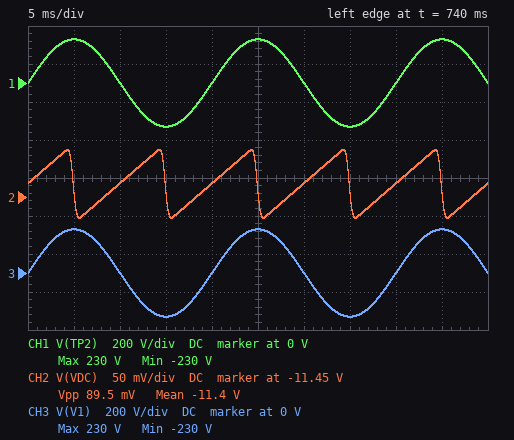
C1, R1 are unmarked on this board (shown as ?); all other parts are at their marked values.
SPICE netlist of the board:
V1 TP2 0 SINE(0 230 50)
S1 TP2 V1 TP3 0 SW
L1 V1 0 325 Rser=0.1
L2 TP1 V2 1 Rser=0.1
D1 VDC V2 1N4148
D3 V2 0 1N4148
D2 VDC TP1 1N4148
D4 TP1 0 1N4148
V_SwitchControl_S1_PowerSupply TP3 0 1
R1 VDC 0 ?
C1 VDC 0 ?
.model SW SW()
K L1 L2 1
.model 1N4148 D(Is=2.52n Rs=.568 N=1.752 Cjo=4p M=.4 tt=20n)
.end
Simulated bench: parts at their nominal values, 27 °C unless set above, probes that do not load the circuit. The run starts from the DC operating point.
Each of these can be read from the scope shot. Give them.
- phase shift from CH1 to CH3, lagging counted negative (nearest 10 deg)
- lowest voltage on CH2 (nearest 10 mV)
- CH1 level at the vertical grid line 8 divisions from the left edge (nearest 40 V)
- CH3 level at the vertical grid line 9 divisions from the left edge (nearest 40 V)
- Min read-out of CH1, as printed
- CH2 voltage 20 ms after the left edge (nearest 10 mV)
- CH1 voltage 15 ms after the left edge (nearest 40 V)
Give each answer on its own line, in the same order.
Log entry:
0 deg
-11.48 V
0 V
240 V
-230 V
-11.43 V
-240 V
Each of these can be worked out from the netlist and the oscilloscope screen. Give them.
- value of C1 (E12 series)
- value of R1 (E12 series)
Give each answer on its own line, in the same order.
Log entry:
33 µF
33 kΩ
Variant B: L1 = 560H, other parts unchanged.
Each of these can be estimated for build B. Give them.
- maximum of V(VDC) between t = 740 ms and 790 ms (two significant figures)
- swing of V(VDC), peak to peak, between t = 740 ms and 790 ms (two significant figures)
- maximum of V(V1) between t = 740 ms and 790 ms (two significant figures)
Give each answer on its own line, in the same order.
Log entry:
-8.4 V
65 mV
230 V
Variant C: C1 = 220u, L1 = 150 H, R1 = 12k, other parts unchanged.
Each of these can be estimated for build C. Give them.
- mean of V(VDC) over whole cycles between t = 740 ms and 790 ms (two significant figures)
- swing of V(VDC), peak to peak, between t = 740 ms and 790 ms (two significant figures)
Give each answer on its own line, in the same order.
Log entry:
-17 V
57 mV
